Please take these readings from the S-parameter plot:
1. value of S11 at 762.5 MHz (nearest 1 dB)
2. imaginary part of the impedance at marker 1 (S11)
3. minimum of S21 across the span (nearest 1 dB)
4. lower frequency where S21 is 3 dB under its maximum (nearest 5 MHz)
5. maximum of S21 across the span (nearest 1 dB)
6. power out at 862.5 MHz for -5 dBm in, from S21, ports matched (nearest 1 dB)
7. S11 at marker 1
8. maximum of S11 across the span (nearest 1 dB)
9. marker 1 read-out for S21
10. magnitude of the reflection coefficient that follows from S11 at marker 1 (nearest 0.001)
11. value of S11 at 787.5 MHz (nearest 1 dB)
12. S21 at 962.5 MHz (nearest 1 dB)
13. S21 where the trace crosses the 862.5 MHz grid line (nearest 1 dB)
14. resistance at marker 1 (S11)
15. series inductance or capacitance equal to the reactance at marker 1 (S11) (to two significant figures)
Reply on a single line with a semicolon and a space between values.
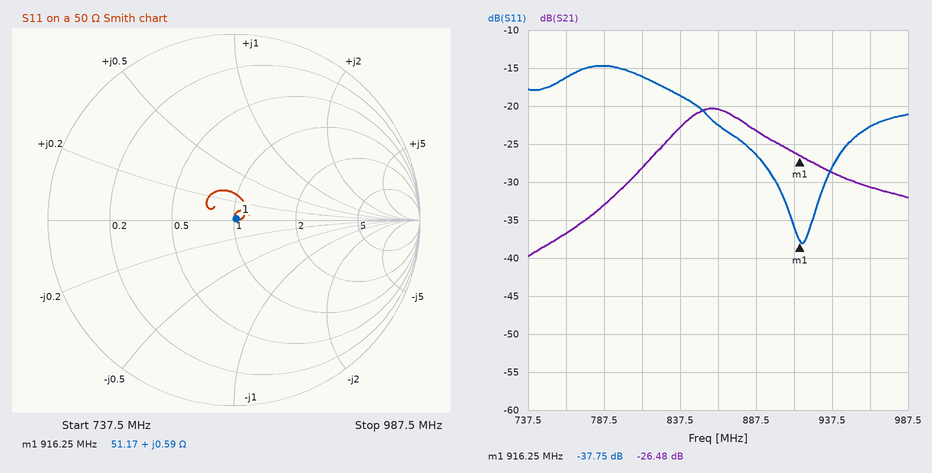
-16 dB; +0.59 Ω; -40 dB; 835 MHz; -20 dB; -25 dBm; -37.75 dB; -15 dB; -26.48 dB; 0.013; -15 dB; -31 dB; -20 dB; 51.17 Ω; 100 pH
